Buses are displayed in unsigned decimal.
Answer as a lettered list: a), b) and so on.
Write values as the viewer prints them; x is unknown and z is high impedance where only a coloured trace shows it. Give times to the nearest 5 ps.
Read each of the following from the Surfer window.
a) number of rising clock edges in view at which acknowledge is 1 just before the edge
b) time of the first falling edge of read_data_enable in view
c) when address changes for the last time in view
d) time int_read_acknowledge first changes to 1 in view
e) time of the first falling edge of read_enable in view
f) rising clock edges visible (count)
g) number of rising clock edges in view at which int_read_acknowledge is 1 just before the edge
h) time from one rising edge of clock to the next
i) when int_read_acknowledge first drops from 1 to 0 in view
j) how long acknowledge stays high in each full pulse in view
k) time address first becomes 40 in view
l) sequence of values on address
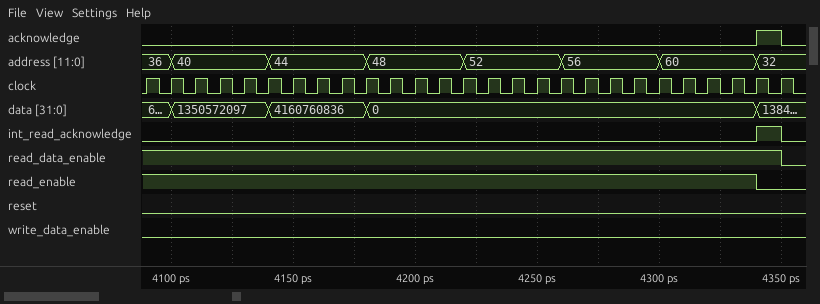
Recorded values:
a) 1
b) 4350 ps
c) 4340 ps
d) 4340 ps
e) 4340 ps
f) 27
g) 1
h) 10 ps
i) 4350 ps
j) 10 ps
k) 4100 ps
l) 36, 40, 44, 48, 52, 56, 60, 32
